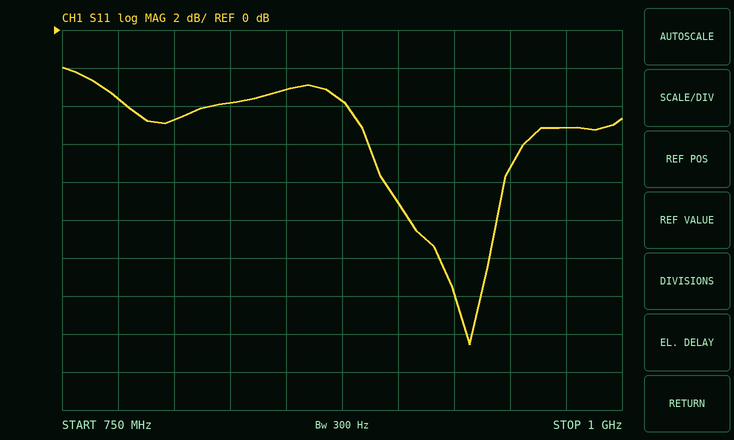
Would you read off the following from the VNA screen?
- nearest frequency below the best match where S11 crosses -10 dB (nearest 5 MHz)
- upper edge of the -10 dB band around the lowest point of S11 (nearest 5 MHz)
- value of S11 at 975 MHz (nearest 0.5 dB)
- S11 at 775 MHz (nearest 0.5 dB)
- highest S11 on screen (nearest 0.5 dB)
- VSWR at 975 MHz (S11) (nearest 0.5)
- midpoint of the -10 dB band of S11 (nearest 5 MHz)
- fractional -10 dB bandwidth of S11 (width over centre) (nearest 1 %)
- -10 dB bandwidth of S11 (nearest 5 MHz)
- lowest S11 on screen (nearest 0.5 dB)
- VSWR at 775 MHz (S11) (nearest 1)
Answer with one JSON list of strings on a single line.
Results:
["905 MHz", "945 MHz", "-5.0 dB", "-3.5 dB", "-2.0 dB", "3.5", "925 MHz", "4 %", "40 MHz", "-16.5 dB", "5"]
